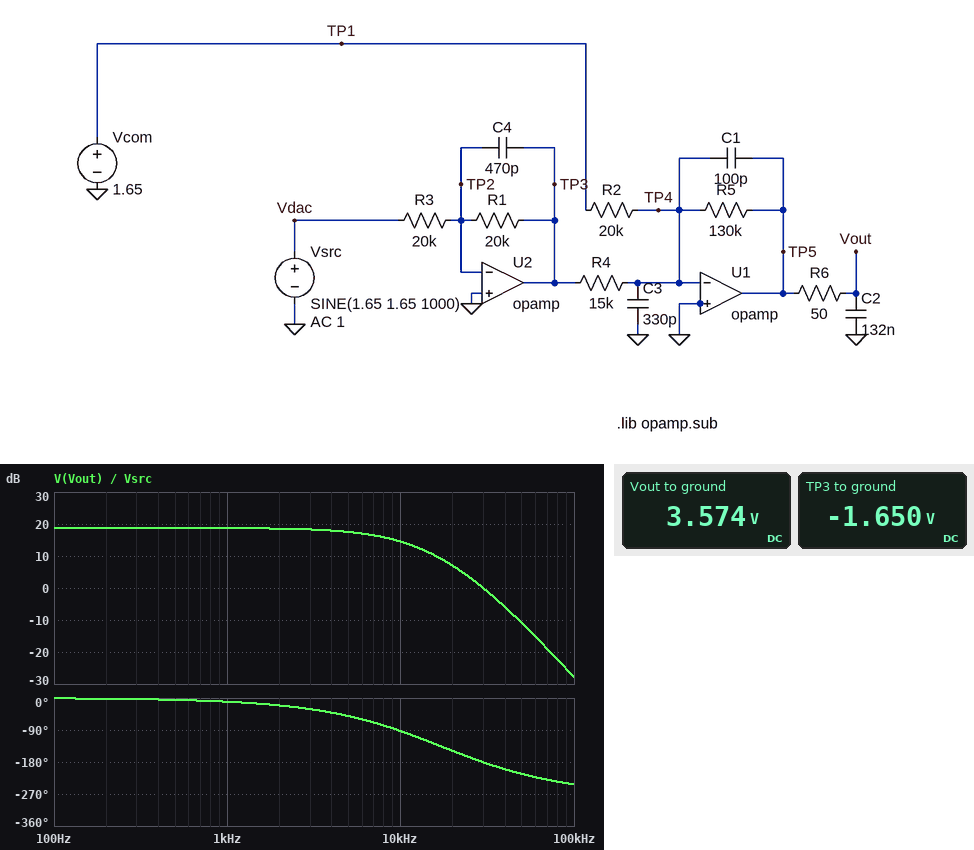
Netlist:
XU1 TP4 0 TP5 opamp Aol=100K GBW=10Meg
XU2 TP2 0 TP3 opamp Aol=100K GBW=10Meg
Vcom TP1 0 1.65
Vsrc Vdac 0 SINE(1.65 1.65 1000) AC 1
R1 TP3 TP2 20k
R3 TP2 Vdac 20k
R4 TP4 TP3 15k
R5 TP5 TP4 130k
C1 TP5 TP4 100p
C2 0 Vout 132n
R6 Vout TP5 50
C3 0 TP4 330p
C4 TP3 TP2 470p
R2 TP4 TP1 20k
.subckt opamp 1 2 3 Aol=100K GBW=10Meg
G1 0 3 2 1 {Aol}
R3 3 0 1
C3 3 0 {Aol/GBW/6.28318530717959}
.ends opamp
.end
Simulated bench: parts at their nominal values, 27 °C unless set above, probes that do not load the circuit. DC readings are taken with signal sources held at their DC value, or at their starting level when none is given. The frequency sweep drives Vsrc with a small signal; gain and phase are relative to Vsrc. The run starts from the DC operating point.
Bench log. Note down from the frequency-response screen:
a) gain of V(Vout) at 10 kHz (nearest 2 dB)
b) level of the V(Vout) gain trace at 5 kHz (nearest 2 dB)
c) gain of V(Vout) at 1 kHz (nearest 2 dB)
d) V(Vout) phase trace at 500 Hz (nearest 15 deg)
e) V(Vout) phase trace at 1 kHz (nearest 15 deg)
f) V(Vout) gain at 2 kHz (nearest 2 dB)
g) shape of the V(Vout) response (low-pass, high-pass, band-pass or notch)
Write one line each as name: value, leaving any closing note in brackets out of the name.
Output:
gain of V(Vout) at 10 kHz: 14 dB
level of the V(Vout) gain trace at 5 kHz: 18 dB
gain of V(Vout) at 1 kHz: 18 dB
V(Vout) phase trace at 500 Hz: 0 deg
V(Vout) phase trace at 1 kHz: -15 deg
V(Vout) gain at 2 kHz: 18 dB
shape of the V(Vout) response: low-pass
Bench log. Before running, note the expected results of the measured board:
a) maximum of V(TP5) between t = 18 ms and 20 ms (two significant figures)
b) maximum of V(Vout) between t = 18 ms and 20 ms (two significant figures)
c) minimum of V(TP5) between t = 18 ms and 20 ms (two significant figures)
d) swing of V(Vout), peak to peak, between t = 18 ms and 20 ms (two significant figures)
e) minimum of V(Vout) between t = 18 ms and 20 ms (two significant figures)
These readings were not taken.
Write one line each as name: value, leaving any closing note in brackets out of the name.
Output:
maximum of V(TP5) between t = 18 ms and 20 ms: 18 V
maximum of V(Vout) between t = 18 ms and 20 ms: 18 V
minimum of V(TP5) between t = 18 ms and 20 ms: -11 V
swing of V(Vout), peak to peak, between t = 18 ms and 20 ms: 28 V
minimum of V(Vout) between t = 18 ms and 20 ms: -11 V
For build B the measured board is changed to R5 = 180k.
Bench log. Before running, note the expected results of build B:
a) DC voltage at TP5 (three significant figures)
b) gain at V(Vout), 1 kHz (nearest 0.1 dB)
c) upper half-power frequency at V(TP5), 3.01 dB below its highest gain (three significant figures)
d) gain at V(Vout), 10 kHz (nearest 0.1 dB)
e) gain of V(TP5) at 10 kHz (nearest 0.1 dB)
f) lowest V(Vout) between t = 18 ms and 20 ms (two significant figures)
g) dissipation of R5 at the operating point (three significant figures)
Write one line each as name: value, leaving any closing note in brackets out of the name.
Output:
DC voltage at TP5: 4.95 V
gain at V(Vout), 1 kHz: 21.5 dB
upper half-power frequency at V(TP5), 3.01 dB below its highest gain: 7.23 kHz
gain at V(Vout), 10 kHz: 15.9 dB
gain of V(TP5) at 10 kHz: 16.6 dB
lowest V(Vout) between t = 18 ms and 20 ms: -15 V
dissipation of R5 at the operating point: 136 µW
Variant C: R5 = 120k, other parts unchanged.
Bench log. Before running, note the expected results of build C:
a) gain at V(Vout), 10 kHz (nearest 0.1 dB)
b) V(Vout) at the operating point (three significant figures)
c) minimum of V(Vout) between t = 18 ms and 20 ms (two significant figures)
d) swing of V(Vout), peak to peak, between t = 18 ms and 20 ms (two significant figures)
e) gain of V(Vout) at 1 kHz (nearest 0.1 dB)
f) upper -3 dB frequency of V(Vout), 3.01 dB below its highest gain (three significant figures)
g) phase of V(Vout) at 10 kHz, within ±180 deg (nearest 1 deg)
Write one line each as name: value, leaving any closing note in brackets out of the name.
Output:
gain at V(Vout), 10 kHz: 14.1 dB
V(Vout) at the operating point: 3.30 V
minimum of V(Vout) between t = 18 ms and 20 ms: -9.8 V
swing of V(Vout), peak to peak, between t = 18 ms and 20 ms: 26 V
gain of V(Vout) at 1 kHz: 18.0 dB
upper -3 dB frequency of V(Vout), 3.01 dB below its highest gain: 8.49 kHz
phase of V(Vout) at 10 kHz, within ±180 deg: -91 deg
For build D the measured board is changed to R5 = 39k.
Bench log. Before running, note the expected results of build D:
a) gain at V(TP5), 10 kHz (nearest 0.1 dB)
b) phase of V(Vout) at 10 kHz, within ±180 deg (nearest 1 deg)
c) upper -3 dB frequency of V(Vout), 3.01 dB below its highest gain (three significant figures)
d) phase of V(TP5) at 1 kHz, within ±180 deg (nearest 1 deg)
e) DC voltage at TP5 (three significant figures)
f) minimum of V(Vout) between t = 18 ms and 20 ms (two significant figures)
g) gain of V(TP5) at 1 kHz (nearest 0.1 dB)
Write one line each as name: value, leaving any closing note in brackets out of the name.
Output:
gain at V(TP5), 10 kHz: 6.7 dB
phase of V(Vout) at 10 kHz, within ±180 deg: -67 deg
upper -3 dB frequency of V(Vout), 3.01 dB below its highest gain: 11.8 kHz
phase of V(TP5) at 1 kHz, within ±180 deg: -5 deg
DC voltage at TP5: 1.07 V
minimum of V(Vout) between t = 18 ms and 20 ms: -3.2 V
gain of V(TP5) at 1 kHz: 8.3 dB
